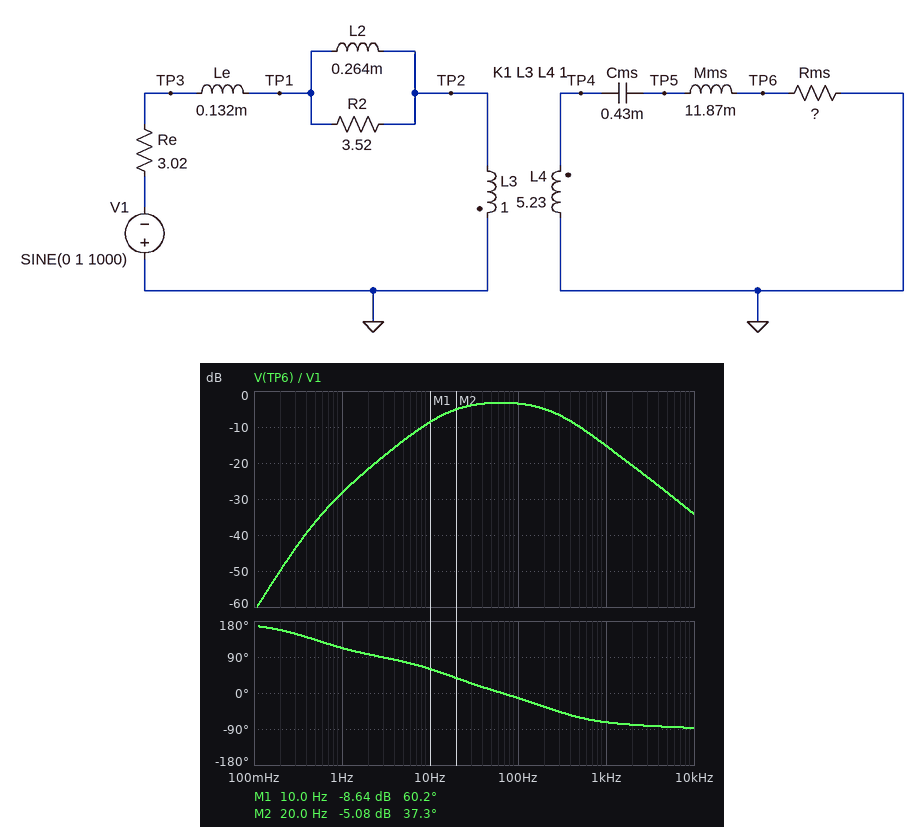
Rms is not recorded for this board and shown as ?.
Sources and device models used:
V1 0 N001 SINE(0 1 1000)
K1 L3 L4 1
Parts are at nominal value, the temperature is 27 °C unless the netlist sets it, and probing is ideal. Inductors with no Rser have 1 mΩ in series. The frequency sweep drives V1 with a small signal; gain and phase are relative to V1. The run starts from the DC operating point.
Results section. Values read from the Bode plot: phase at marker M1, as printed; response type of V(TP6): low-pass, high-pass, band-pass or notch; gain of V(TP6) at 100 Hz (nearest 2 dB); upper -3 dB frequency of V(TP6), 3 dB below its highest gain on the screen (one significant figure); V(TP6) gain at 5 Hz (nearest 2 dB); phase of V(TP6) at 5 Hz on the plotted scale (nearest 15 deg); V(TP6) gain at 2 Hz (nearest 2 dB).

60.2 deg
band-pass
-4 dB
300 Hz
-14 dB
75 deg
-22 dB
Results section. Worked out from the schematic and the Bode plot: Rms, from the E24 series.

6.8 Ω
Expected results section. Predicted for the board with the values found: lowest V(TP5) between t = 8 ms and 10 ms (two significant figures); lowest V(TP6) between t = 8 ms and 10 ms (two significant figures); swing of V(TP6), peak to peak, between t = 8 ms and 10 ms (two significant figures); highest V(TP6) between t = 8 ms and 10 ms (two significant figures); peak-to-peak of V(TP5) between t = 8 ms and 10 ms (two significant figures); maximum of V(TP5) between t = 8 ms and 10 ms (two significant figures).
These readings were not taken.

-1.9 V
-180 mV
350 mV
170 mV
3.8 V
1.9 V
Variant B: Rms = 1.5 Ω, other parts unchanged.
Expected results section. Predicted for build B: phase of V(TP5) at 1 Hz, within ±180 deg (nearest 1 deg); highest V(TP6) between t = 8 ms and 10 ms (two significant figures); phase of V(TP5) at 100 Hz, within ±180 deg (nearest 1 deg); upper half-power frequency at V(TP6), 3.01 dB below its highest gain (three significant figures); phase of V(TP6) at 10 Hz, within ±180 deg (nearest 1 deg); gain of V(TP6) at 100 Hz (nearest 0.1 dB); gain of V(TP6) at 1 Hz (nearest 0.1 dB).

116 deg
37 mV
62 deg
215 Hz
67 deg
-14.4 dB
-41.4 dB
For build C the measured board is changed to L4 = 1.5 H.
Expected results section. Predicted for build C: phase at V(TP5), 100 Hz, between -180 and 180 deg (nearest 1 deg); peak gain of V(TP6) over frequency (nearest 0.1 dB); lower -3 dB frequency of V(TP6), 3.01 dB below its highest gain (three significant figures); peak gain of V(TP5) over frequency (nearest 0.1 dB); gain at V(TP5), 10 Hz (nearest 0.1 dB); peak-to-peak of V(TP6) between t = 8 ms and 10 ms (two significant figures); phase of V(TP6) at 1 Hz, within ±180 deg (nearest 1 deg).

28 deg
-2.7 dB
27.3 Hz
1.6 dB
-13.1 dB
210 mV
114 deg
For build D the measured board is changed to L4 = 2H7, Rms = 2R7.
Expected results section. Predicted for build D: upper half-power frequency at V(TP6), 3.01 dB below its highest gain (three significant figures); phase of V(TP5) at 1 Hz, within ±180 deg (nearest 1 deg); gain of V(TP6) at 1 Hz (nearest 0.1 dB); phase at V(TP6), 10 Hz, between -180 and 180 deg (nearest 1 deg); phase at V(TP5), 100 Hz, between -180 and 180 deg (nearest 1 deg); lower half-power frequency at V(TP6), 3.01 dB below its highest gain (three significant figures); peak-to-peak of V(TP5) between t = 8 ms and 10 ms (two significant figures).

161 Hz
116 deg
-39.3 dB
76 deg
48 deg
27.9 Hz
3.0 V
